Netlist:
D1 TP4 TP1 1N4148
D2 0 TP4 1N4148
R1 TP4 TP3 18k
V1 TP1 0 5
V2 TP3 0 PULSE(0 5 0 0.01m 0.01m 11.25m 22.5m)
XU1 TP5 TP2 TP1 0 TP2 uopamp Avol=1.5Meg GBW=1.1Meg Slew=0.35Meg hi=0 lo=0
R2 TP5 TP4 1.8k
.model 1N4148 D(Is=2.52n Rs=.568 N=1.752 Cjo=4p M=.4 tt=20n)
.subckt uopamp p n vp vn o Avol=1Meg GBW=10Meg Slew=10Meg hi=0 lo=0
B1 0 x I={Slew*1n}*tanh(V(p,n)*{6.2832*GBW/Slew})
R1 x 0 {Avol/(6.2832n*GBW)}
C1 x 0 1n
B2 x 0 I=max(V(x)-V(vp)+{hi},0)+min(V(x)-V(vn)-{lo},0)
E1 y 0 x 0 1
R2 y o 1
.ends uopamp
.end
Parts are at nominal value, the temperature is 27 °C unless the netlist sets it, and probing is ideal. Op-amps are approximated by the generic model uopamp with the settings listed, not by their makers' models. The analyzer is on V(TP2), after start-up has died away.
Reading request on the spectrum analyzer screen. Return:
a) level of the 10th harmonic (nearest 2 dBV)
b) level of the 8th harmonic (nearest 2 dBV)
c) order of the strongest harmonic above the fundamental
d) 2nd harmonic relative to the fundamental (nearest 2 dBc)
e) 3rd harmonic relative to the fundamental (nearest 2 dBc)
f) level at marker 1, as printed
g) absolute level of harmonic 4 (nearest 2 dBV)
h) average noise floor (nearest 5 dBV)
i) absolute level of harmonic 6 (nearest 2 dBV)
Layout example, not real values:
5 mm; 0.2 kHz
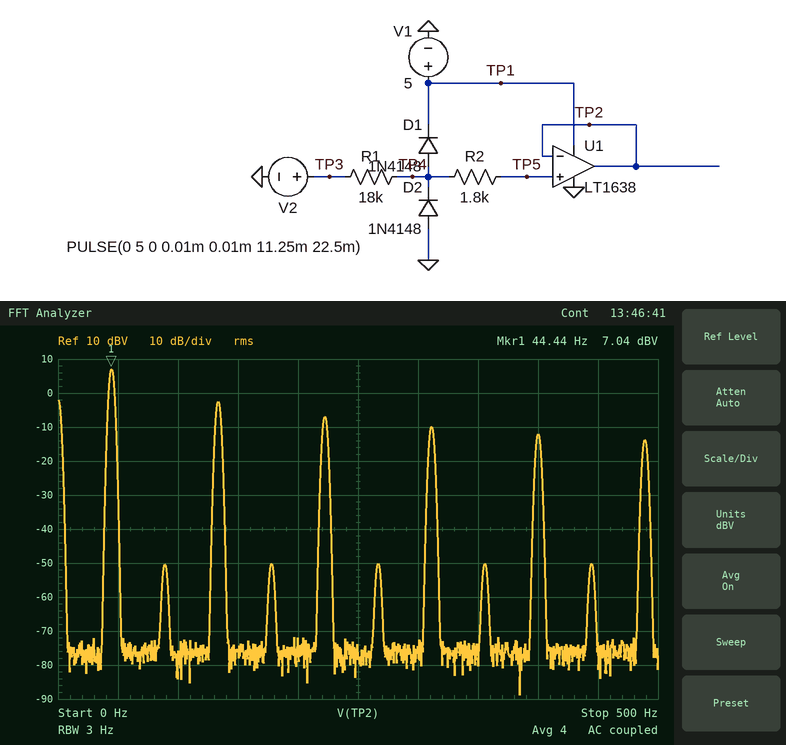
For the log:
-50 dBV; -50 dBV; 3; -58 dBc; -10 dBc; 7.04 dBV; -50 dBV; -75 dBV; -50 dBV
